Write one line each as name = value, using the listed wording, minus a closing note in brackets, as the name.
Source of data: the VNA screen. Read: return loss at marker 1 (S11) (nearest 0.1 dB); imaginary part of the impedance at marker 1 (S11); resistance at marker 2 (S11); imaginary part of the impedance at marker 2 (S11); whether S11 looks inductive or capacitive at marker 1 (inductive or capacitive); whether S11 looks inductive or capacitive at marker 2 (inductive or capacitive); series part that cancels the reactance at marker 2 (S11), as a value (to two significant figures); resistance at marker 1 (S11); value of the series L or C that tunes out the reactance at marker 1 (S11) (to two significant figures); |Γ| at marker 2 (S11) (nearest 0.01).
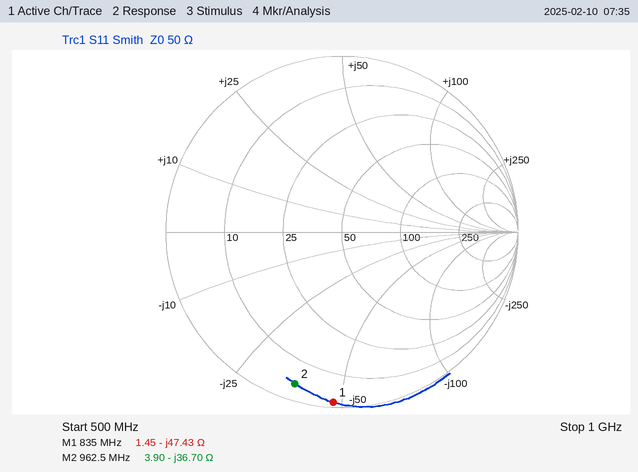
return loss at marker 1 (S11) = 0.3 dB
imaginary part of the impedance at marker 1 = -47.43 Ω
resistance at marker 2 = 3.90 Ω
imaginary part of the impedance at marker 2 = -36.70 Ω
whether S11 looks inductive or capacitive at marker 1 = capacitive
whether S11 looks inductive or capacitive at marker 2 = capacitive
series part that cancels the reactance at marker 2 (S11), as a value = 6.1 nH
resistance at marker 1 = 1.45 Ω
value of the series L or C that tunes out the reactance at marker 1 (S11) = 9.0 nH
|Γ| at marker 2 (S11) = 0.90
